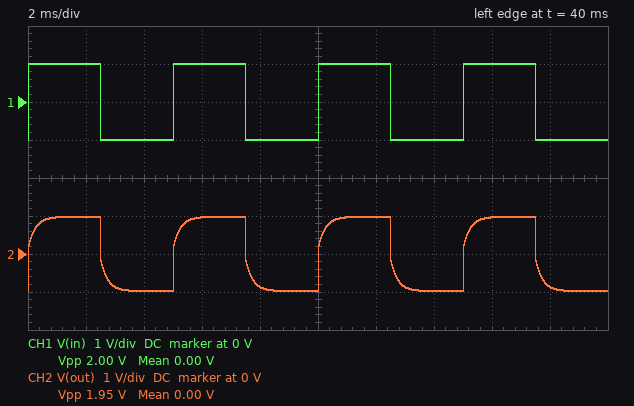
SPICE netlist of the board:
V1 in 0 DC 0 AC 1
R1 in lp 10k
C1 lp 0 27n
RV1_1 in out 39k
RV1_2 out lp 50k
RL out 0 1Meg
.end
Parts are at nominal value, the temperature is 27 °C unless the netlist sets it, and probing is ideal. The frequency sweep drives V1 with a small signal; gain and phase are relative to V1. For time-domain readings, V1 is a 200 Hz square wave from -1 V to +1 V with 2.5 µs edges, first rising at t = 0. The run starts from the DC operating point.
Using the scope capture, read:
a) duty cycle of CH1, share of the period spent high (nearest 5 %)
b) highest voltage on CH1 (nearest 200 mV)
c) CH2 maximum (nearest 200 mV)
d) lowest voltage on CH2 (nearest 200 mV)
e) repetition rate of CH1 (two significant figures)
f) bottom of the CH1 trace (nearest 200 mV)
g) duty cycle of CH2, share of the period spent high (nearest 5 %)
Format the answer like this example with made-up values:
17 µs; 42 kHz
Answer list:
50 %; 1.0 V; 1.0 V; -1.0 V; 200 Hz; -1.0 V; 50 %
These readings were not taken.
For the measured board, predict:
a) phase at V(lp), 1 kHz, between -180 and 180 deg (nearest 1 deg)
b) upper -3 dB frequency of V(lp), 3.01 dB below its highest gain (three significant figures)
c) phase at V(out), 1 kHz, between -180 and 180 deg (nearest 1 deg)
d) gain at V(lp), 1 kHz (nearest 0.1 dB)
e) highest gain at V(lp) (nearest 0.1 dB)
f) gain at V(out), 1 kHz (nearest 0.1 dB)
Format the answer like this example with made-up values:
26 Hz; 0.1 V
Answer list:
-57 deg; 657 Hz; -16 deg; -5.2 dB; 0 dB; -3.0 dB
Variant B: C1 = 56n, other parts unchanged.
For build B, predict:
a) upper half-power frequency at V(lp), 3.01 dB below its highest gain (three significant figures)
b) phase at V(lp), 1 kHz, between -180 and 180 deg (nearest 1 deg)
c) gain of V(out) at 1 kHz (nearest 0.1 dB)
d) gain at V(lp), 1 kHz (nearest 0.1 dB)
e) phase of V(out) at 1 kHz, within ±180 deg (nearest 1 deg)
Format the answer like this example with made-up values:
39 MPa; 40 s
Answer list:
317 Hz; -72 deg; -4.4 dB; -10.4 dB; -12 deg
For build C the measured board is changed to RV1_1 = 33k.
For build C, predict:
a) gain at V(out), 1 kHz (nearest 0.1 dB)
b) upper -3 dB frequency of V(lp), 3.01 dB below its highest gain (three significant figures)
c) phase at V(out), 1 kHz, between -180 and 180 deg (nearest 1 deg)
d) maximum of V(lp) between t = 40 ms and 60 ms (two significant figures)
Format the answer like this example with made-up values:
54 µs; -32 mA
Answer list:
-2.7 dB; 661 Hz; -14 deg; 1.0 V
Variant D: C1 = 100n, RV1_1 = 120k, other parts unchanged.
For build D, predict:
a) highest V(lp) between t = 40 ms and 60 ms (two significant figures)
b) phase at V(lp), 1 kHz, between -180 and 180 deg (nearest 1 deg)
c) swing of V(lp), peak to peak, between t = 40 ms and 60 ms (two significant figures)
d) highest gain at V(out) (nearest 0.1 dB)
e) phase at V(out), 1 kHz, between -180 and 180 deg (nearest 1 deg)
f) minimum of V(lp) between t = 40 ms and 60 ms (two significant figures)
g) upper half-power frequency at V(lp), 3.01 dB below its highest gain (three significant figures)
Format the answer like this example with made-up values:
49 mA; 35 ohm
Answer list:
860 mV; -80 deg; 1.7 V; -0.3 dB; -20 deg; -860 mV; 169 Hz
